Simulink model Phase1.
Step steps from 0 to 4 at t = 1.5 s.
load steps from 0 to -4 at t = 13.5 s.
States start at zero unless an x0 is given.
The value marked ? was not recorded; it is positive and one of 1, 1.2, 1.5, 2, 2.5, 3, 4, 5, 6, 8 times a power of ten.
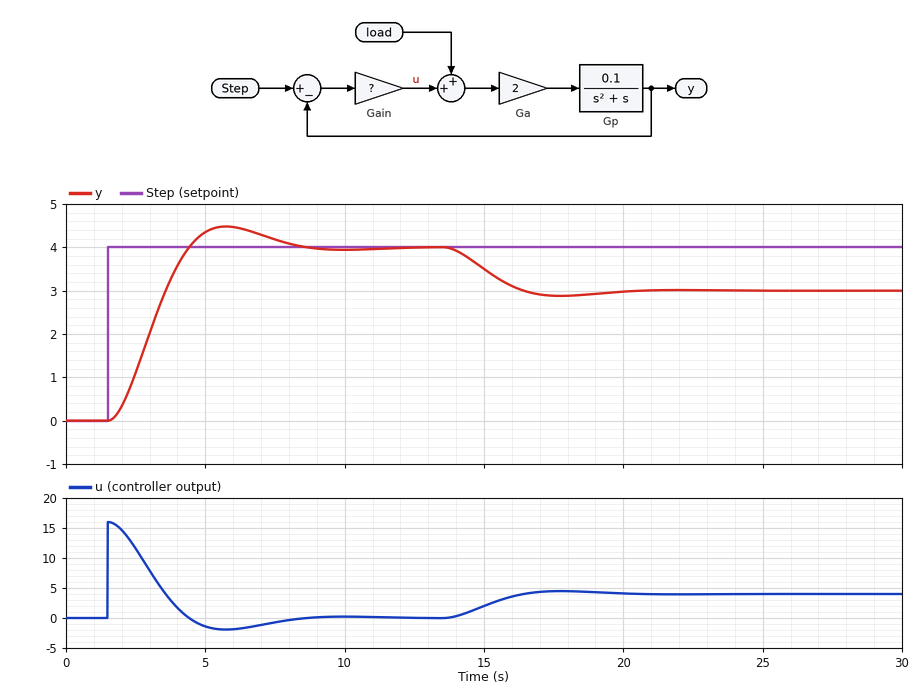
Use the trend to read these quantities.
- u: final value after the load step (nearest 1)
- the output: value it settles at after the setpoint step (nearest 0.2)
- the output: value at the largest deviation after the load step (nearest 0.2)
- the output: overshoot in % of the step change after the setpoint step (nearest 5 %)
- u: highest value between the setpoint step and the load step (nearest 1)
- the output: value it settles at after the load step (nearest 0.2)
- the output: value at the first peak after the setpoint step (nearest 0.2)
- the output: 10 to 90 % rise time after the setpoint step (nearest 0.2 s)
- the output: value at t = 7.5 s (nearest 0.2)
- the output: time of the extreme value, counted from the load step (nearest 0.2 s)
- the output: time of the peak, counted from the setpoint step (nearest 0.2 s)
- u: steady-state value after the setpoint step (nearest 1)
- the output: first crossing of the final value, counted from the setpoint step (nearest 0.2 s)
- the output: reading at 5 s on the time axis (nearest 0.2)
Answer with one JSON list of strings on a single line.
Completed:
["4", "4.0", "2.8", "10 %", "16", "3.0", "4.4", "2.0 s", "4.2", "4.2 s", "4.2 s", "0", "3.0 s", "4.4"]
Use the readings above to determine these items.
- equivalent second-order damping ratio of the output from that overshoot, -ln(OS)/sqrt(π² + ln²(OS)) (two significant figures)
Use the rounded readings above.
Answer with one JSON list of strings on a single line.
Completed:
["0.59"]
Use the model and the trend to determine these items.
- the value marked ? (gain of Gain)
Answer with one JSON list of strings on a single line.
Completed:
["4"]
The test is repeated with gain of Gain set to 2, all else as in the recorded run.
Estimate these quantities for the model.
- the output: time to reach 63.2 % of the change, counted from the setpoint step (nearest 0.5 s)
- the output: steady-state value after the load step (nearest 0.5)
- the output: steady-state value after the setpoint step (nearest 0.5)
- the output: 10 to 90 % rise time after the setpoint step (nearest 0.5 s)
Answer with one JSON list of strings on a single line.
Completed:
["3.0 s", "2.0", "4.0", "4.0 s"]
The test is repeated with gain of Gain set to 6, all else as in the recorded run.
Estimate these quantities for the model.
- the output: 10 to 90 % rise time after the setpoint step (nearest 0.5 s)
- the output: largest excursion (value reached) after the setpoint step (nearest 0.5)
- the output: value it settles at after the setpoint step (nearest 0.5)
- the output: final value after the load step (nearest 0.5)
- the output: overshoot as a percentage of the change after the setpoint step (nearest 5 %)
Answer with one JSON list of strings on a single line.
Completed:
["1.5 s", "5.0", "4.0", "3.5", "20 %"]
